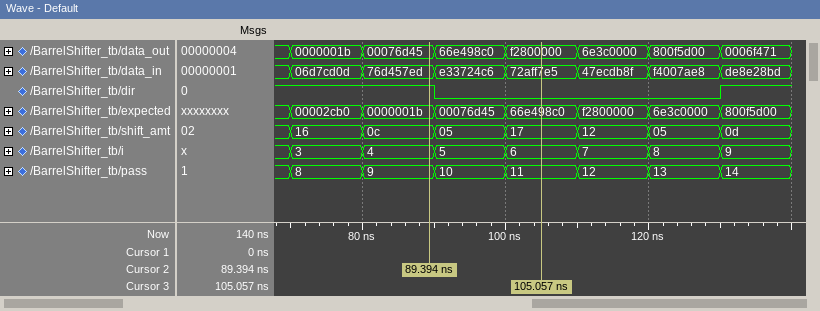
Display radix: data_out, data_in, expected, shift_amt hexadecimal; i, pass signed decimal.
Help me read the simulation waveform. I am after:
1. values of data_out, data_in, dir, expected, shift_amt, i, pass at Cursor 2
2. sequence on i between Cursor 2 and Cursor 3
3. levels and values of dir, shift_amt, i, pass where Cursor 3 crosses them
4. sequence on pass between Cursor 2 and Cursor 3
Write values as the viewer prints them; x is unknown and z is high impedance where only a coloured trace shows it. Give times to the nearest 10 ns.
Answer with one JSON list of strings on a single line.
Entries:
["data_out=00076d45, data_in=76d457ed, dir=1, expected=0000001b, shift_amt=0c, i=4, pass=9", "4, 5, 6", "dir=0, shift_amt=17, i=6, pass=11", "9, 10, 11"]
